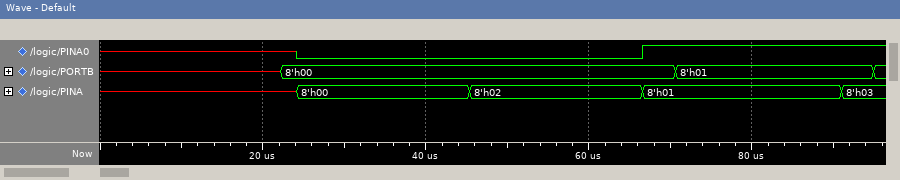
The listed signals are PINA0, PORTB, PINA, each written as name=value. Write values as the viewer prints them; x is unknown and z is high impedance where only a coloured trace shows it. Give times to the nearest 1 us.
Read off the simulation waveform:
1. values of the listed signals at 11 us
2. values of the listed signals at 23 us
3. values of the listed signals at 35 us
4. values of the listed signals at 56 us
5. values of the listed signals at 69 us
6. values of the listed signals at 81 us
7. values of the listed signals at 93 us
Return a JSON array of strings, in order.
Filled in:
["PINA0=x, PORTB=x, PINA=x", "PINA0=x, PORTB=8'h00, PINA=x", "PINA0=0, PORTB=8'h00, PINA=8'h00", "PINA0=0, PORTB=8'h00, PINA=8'h02", "PINA0=1, PORTB=8'h00, PINA=8'h01", "PINA0=1, PORTB=8'h01, PINA=8'h01", "PINA0=1, PORTB=8'h01, PINA=8'h03"]
